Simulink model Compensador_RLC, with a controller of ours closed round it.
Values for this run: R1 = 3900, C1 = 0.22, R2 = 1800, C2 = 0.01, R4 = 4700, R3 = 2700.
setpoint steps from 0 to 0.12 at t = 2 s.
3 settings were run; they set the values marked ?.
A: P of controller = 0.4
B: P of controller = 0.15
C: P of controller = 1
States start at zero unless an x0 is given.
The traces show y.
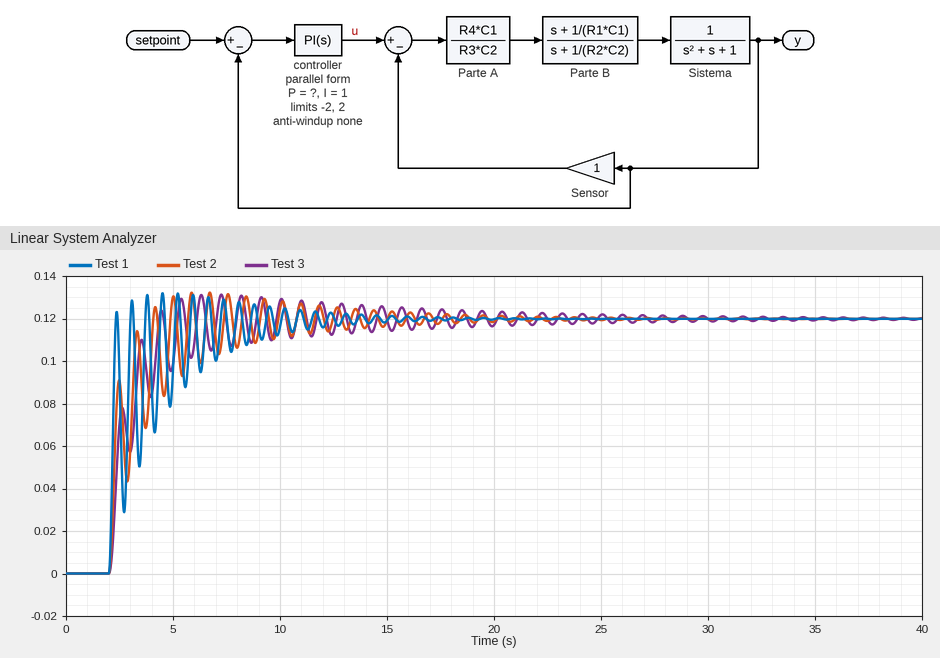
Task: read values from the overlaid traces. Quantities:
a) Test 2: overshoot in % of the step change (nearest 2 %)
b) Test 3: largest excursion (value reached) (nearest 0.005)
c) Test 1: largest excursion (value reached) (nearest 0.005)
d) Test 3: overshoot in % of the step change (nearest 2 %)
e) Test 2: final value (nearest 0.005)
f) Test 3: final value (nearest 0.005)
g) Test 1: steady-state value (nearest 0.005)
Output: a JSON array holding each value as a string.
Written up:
["10 %", "0.130", "0.130", "10 %", "0.120", "0.120", "0.120"]
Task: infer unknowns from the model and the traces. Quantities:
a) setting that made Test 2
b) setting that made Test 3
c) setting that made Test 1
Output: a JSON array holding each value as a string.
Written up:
["A", "B", "C"]
